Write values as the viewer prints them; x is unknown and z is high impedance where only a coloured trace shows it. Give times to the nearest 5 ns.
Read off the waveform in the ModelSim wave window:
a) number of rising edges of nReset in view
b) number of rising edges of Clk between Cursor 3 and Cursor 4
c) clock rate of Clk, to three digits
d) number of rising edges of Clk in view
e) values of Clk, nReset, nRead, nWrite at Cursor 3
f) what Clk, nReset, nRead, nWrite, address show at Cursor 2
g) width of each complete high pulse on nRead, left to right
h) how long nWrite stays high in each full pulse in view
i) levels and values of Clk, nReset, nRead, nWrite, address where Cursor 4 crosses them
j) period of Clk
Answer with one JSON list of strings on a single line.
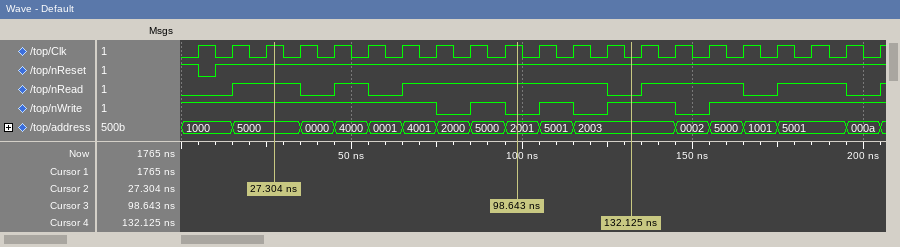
["1", "3", "100 MHz", "21", "Clk=1, nReset=1, nRead=1, nWrite=0", "Clk=1, nReset=1, nRead=1, nWrite=1, address=5000", "20 ns, 10 ns, 60 ns, 30 ns, 20 ns", "10 ns, 10 ns, 20 ns", "Clk=0, nReset=1, nRead=0, nWrite=1, address=2003", "10 ns"]
